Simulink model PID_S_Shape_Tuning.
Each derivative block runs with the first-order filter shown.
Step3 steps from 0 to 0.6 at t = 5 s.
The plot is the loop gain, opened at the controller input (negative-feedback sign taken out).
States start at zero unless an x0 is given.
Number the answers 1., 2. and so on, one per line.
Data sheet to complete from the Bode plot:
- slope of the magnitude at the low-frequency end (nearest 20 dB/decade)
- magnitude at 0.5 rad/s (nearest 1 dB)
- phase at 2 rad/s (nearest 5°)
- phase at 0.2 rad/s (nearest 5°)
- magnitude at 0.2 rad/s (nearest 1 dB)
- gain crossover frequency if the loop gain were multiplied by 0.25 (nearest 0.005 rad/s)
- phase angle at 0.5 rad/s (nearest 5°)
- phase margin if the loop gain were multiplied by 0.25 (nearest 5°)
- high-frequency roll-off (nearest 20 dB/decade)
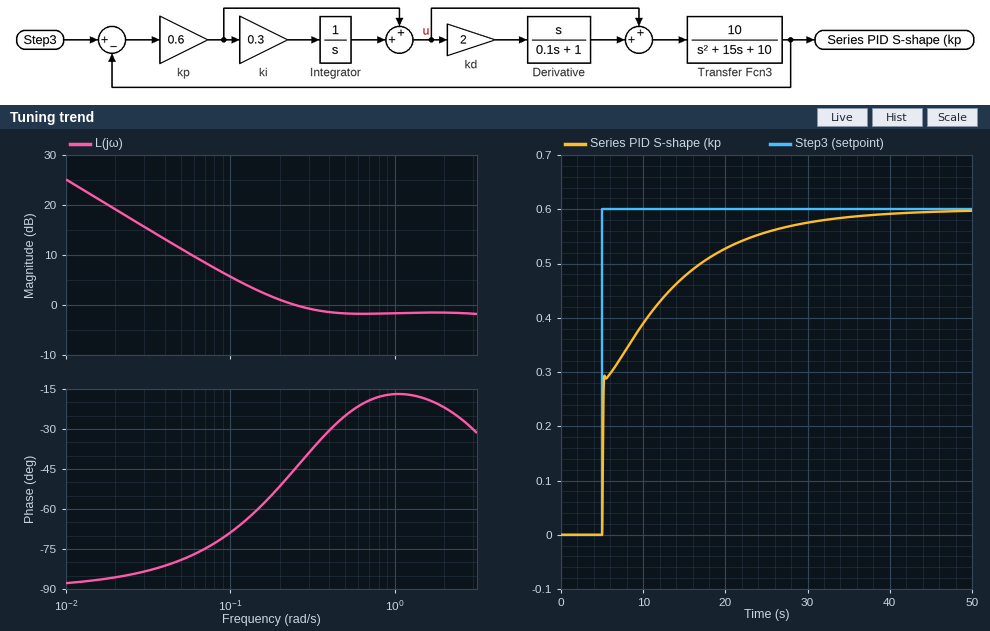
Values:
1. -20 dB/decade
2. -2 dB
3. -20°
4. -50°
5. 1 dB
6. 0.045 rad/s
7. -25°
8. 100°
9. 0 dB/decade
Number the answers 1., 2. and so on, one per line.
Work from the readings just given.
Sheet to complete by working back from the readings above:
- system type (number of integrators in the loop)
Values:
1. 1
